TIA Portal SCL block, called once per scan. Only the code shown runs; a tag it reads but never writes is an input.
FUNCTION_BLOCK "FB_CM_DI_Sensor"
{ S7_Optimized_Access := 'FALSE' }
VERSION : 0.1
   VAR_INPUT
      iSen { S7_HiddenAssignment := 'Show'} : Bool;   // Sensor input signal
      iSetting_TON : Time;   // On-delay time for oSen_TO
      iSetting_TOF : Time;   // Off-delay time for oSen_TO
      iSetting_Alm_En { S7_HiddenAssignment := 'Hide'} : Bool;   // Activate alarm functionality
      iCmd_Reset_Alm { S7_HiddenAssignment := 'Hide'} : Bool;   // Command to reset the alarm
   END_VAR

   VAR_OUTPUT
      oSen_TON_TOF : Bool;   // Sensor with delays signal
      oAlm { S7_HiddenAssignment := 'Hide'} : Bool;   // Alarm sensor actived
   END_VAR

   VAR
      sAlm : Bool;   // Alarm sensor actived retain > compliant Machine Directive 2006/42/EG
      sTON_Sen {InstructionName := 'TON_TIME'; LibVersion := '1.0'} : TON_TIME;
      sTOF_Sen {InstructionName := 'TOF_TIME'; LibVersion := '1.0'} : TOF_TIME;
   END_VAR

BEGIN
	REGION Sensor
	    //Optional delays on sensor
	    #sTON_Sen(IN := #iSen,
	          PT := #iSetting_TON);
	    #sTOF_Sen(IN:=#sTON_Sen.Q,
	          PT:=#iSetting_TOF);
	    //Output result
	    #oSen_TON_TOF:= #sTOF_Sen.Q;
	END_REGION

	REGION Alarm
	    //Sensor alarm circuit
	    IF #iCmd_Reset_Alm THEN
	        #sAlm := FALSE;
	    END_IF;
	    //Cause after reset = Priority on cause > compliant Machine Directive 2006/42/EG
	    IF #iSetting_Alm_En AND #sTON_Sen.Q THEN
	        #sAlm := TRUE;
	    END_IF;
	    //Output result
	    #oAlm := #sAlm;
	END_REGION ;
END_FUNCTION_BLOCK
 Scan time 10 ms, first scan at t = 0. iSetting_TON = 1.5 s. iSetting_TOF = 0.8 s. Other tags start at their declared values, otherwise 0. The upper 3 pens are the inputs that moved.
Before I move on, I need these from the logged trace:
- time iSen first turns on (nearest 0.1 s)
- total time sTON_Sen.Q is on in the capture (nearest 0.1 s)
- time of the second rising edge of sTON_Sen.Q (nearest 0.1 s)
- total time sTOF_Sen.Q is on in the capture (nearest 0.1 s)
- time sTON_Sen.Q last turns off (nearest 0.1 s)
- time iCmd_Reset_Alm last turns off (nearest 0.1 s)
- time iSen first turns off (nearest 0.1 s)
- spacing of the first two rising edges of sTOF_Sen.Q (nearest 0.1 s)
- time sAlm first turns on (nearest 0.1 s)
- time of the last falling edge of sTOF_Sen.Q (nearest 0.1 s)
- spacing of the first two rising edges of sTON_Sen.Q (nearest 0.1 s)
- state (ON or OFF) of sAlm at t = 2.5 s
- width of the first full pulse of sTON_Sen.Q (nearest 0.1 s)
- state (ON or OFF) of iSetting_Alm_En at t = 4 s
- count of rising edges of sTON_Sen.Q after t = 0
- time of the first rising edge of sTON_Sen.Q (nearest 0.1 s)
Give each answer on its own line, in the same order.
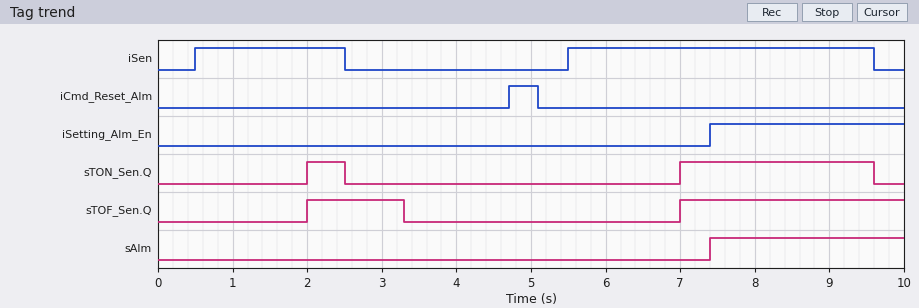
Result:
0.5 s
3.1 s
7.0 s
4.3 s
9.6 s
5.1 s
2.5 s
5.0 s
7.4 s
3.3 s
5.0 s
OFF
0.5 s
OFF
2
2.0 s
